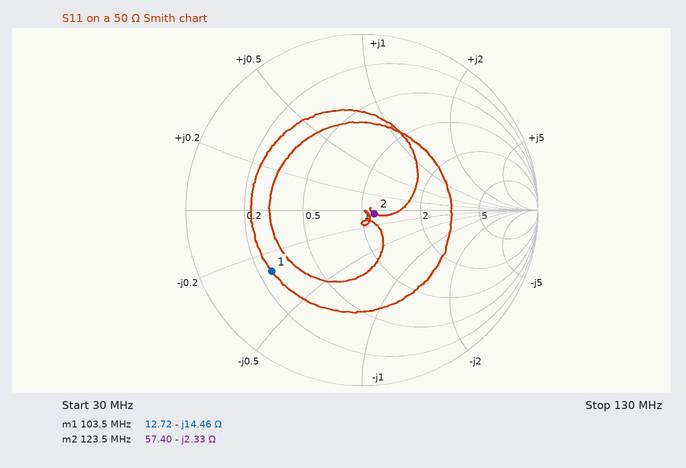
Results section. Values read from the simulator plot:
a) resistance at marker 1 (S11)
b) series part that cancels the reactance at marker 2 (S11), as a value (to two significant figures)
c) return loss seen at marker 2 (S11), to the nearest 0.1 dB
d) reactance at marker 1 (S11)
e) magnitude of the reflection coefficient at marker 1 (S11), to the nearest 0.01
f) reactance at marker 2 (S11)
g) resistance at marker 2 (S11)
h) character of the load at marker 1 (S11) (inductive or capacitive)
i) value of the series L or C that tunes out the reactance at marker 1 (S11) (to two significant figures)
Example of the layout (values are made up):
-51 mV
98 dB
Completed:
12.72 Ω
3.0 nH
22.8 dB
-14.46 Ω
0.62
-2.33 Ω
57.40 Ω
capacitive
22 nH
